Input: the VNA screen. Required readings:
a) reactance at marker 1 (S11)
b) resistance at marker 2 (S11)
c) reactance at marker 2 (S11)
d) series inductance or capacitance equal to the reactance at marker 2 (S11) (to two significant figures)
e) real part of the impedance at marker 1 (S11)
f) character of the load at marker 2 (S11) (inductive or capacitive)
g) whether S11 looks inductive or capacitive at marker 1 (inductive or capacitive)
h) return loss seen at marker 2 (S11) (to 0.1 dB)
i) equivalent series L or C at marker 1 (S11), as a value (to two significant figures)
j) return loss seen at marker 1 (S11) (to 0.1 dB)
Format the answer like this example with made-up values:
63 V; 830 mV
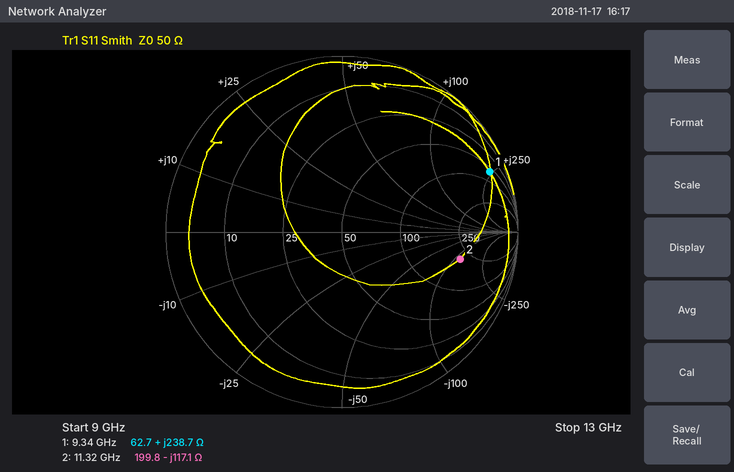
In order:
+238.7 Ω; 199.8 Ω; -117.1 Ω; 120 fF; 62.7 Ω; capacitive; inductive; 3.2 dB; 4.1 nH; 0.9 dB
